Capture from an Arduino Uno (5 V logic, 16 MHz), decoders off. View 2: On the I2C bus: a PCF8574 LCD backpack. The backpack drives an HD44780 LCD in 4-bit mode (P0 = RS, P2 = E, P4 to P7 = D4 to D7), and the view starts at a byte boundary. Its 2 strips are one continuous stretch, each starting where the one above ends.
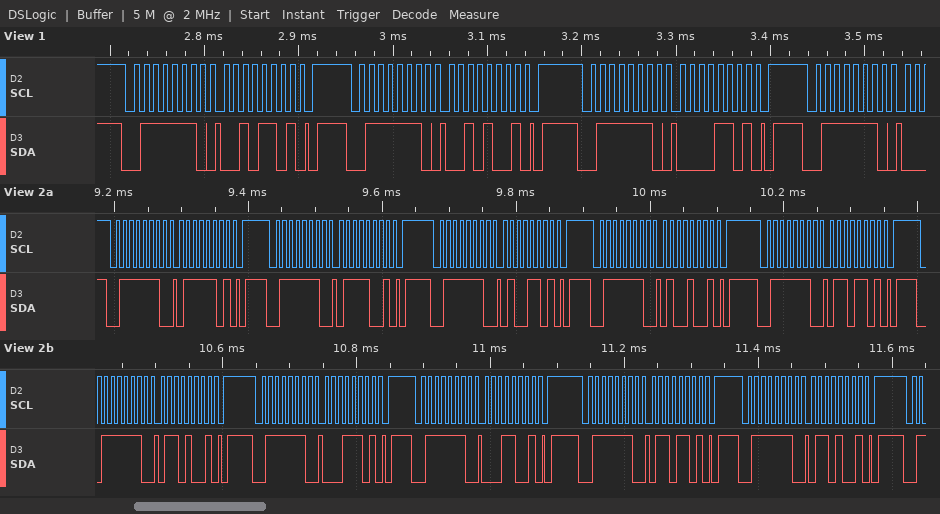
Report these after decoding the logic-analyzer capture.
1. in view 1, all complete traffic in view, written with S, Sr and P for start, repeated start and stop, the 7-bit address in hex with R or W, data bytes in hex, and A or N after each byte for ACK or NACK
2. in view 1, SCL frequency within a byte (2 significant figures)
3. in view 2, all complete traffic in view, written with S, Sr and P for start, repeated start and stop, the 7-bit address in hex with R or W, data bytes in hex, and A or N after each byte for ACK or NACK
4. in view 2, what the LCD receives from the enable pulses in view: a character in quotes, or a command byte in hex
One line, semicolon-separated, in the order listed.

S 3FW A 2D A P S 3FW A 29 A P S 3FW A 0D A P S 3FW A; 100 kHz; S 3FW A 7D A P S 3FW A 79 A P S 3FW A 4D A P S 3FW A 49 A P S 3FW A 6D A P S 3FW A 69 A P S 3FW A 1D A P S 3FW A 19 A P S 3FW A 6D A P S 3FW A 69 A P; 't' 'a'
